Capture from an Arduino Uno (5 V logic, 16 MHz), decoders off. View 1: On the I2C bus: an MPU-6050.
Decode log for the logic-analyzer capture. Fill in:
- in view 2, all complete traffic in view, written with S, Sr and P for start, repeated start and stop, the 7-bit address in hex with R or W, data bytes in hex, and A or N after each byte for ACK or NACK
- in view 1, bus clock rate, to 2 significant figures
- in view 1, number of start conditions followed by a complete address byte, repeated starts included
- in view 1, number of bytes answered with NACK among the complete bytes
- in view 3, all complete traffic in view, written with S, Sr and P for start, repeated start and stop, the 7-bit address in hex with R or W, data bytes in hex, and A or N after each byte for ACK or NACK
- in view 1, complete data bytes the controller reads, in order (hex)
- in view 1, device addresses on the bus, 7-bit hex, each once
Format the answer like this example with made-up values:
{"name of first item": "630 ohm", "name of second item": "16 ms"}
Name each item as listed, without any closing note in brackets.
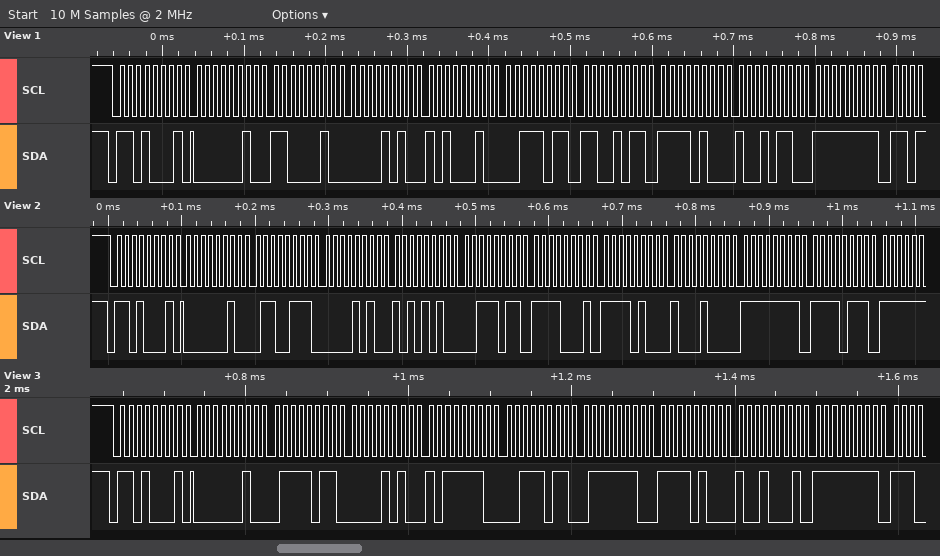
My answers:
{"in view 2, all complete traffic in view, written with S, Sr and P for start, repeated start and stop, the 7-bit address in hex with R or W, data bytes in hex, and A or N after each byte for ACK or NACK": "S 68R A 02 A 67 A 0A A AA A 3B A F1 A F4 A 88 A FF A F7 A", "in view 1, bus clock rate, to 2 significant figures": "100 kHz", "in view 1, number of start conditions followed by a complete address byte, repeated starts included": "1", "in view 1, number of bytes answered with NACK among the complete bytes": "0", "in view 3, all complete traffic in view, written with S, Sr and P for start, repeated start and stop, the 7-bit address in hex with R or W, data bytes in hex, and A or N after each byte for ACK or NACK": "S 68R A 02 A 7B A 0A A BE A 3B A 7E A F4 A 91 A FF A", "in view 1, complete data bytes the controller reads, in order": "02 C2 0A A2 3B CB F4 96 FF", "in view 1, device addresses on the bus, 7-bit hex, each once": "0x68"}
